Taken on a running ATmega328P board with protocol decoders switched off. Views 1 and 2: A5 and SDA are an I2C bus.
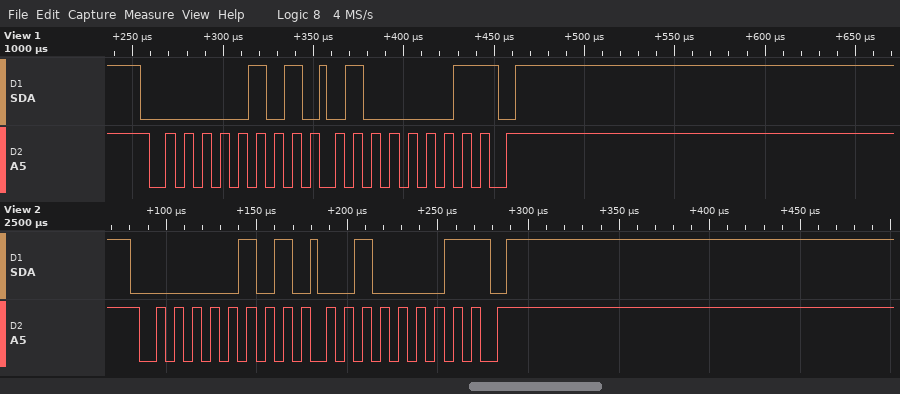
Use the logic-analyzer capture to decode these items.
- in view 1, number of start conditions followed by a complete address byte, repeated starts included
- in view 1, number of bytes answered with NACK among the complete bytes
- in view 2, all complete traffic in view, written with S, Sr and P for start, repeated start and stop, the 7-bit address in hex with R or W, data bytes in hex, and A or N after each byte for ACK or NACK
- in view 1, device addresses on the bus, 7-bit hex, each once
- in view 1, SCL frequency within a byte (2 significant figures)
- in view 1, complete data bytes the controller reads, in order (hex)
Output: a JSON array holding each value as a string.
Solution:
["1", "1", "S 02R A 21 N P", "0x02", "100 kHz", "41"]
